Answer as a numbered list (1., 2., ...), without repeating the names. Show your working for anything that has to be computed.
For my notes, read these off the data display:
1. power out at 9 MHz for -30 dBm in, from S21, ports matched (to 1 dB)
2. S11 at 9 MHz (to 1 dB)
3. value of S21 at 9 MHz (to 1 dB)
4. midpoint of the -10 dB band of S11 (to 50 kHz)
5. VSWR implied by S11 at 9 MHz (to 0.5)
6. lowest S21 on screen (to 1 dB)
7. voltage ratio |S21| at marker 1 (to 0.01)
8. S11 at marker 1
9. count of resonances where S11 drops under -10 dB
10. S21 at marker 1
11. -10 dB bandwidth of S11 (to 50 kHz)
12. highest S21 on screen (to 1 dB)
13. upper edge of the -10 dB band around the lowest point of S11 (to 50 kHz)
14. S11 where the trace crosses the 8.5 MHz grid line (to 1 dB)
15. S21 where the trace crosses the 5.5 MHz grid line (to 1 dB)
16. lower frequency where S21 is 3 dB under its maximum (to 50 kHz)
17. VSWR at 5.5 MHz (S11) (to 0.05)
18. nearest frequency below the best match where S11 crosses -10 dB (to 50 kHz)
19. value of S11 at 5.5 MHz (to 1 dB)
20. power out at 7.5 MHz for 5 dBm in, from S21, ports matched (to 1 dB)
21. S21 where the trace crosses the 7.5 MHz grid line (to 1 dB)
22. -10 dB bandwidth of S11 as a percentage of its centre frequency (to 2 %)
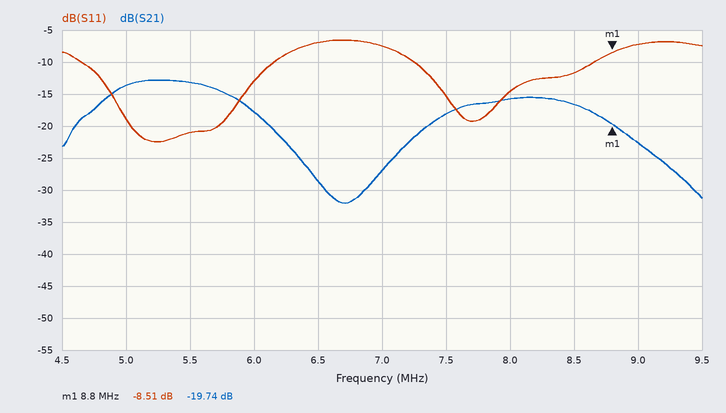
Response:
1. -30 dBm + (-23 dB) = -53 dBm
2. -7 dB
3. -23 dB
4. 5.40 MHz
5. |Γ| = 10^(-7/20) = 0.4467; VSWR = (1 + 0.4467)/(1 − 0.4467) ≈ 2.61, so 2.5 to the nearest 0.5
6. -32 dB
7. 10^(-19.74/20) ≈ 0.10
8. -8.51 dB
9. 2
10. -19.74 dB
11. 6.15 MHz − 4.65 MHz = 1.50 MHz
12. -13 dB
13. 6.15 MHz
14. -12 dB
15. -13 dB
16. 4.85 MHz
17. |Γ| = 10^(-21/20) = 0.0891; VSWR = (1 + 0.0891)/(1 − 0.0891) ≈ 1.20
18. 4.65 MHz
19. -21 dB
20. 5 dBm + (-18 dB) = -13 dBm
21. -18 dB
22. 1.5 MHz / 5.4 MHz ≈ 28 %
